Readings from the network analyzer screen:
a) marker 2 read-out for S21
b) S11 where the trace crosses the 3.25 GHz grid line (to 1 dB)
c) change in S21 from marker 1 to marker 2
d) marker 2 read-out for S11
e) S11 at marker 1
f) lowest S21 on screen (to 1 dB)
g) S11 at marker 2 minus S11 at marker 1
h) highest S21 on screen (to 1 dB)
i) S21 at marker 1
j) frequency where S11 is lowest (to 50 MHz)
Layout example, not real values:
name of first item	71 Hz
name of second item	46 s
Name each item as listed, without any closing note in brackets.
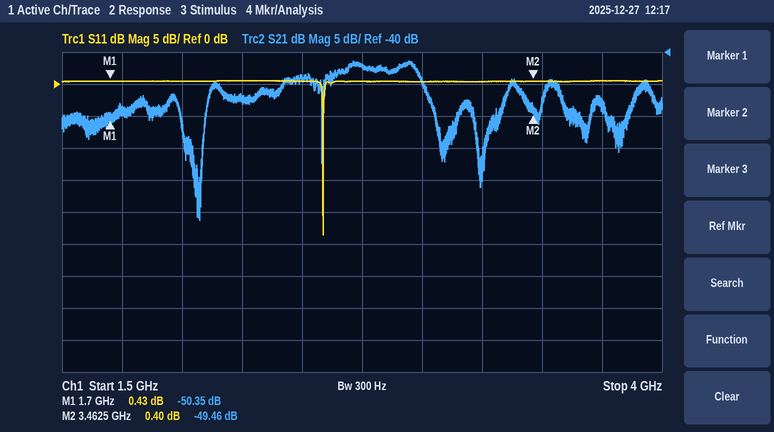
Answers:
marker 2 read-out for S21	-49.46 dB
S11 where the trace crosses the 3.25 GHz grid line	0 dB
change in S21 from marker 1 to marker 2	0.89 dB
marker 2 read-out for S11	0.40 dB
S11 at marker 1	0.43 dB
lowest S21 on screen	-66 dB
S11 at marker 2 minus S11 at marker 1	-0.03 dB
highest S21 on screen	-41 dB
S21 at marker 1	-50.35 dB
frequency where S11 is lowest	2.60 GHz
